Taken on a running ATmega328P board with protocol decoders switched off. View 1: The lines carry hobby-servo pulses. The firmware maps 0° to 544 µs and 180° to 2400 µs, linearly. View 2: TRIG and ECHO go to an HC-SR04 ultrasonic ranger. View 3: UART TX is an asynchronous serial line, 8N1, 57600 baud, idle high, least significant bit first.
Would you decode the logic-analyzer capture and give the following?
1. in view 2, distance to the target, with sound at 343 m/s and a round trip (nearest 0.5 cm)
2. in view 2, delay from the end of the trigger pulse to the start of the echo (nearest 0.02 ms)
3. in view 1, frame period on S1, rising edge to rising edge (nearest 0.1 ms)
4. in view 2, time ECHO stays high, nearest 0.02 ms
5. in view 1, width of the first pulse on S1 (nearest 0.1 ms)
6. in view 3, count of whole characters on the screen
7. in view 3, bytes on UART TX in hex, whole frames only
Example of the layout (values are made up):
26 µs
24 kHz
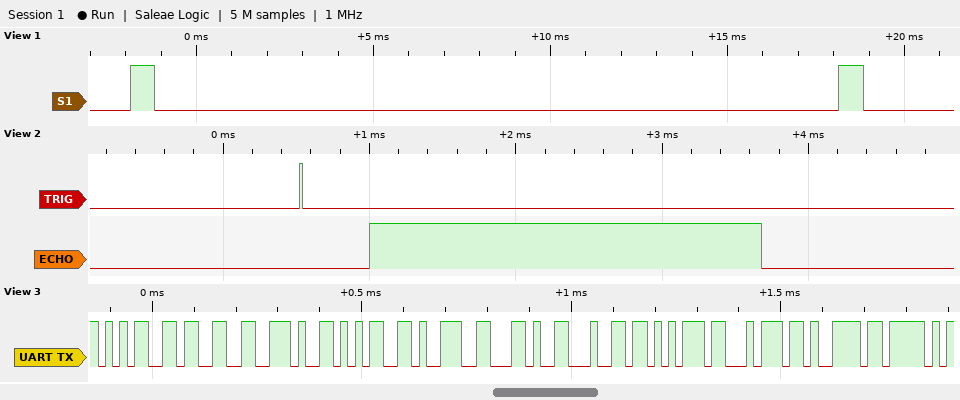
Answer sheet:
46 cm
0.46 ms
20.0 ms
2.68 ms
0.7 ms
11
35 33 2E 35 39 2C 64 75 74 79 5F
